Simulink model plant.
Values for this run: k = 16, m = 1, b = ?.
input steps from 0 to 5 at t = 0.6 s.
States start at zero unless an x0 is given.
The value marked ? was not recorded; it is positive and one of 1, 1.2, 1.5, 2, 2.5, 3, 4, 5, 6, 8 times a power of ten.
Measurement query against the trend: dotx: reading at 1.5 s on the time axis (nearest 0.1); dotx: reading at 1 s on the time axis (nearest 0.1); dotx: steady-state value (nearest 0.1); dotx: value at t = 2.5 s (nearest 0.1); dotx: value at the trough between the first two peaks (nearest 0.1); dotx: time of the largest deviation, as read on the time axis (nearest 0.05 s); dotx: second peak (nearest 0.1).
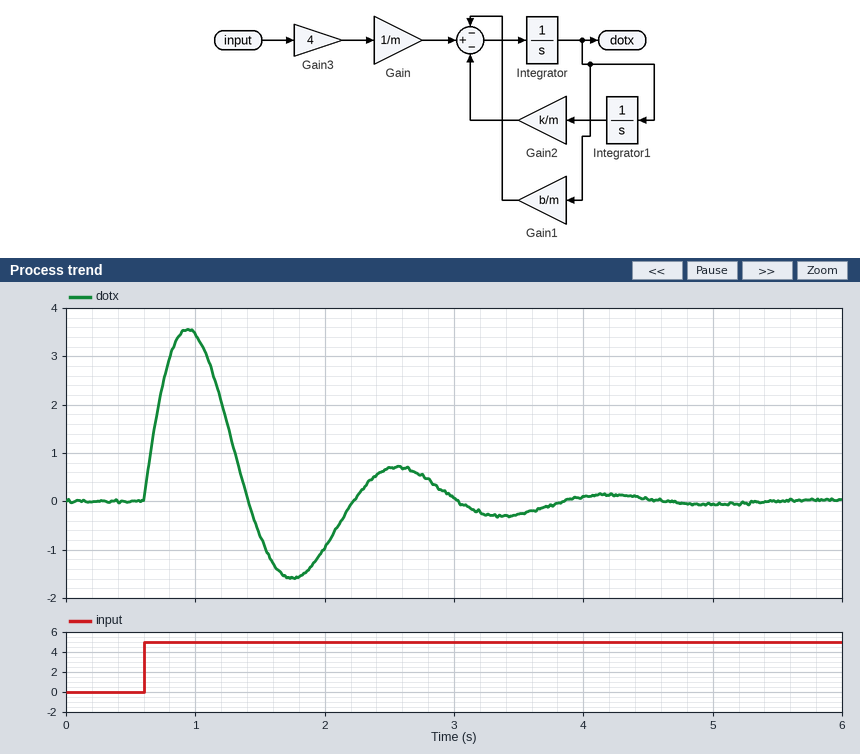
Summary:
-0.7
3.5
0.0
0.7
-1.6
0.95 s
0.7
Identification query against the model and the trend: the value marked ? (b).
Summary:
2
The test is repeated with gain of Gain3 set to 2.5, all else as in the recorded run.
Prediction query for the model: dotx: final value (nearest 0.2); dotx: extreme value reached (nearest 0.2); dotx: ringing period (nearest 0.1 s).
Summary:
0.0
2.2
1.6 s
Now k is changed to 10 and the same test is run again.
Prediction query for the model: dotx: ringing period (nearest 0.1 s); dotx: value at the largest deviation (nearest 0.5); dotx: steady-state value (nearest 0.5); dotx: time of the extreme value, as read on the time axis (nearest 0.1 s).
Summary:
2.1 s
4.0
0.0
1.0 s
